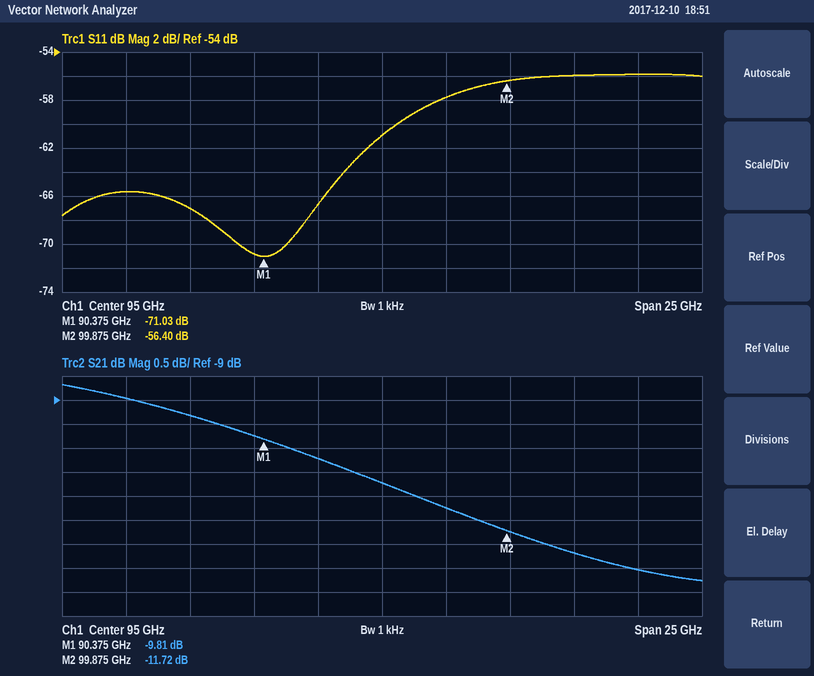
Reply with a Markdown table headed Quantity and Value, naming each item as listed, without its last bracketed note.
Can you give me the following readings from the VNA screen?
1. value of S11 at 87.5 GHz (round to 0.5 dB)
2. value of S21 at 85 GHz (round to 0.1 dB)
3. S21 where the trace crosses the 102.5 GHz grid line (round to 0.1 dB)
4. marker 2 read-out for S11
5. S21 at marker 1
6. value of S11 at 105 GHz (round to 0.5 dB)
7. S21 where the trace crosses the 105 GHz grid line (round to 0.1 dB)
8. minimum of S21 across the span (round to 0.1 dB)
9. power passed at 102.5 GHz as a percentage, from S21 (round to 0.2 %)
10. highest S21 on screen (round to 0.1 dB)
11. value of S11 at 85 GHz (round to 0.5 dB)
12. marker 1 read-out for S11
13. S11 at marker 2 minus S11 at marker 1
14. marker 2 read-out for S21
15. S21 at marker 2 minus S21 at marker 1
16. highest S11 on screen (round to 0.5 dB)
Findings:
| Quantity | Value |
|---|---|
| value of S11 at 87.5 GHz | -67.0 dB |
| value of S21 at 85 GHz | -9.0 dB |
| S21 where the trace crosses the 102.5 GHz grid line | -12.2 dB |
| marker 2 read-out for S11 | -56.40 dB |
| S21 at marker 1 | -9.81 dB |
| value of S11 at 105 GHz | -56.0 dB |
| S21 where the trace crosses the 105 GHz grid line | -12.5 dB |
| minimum of S21 across the span | -12.8 dB |
| power passed at 102.5 GHz as a percentage, from S21 | 6.0 % |
| highest S21 on screen | -8.7 dB |
| value of S11 at 85 GHz | -65.5 dB |
| marker 1 read-out for S11 | -71.03 dB |
| S11 at marker 2 minus S11 at marker 1 | 14.63 dB |
| marker 2 read-out for S21 | -11.72 dB |
| S21 at marker 2 minus S21 at marker 1 | -1.91 dB |
| highest S11 on screen | -56.0 dB |
